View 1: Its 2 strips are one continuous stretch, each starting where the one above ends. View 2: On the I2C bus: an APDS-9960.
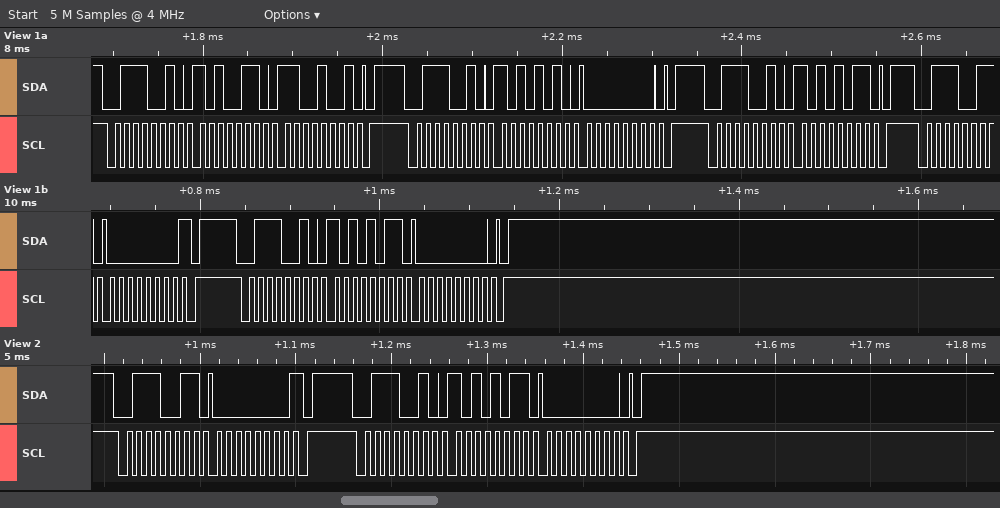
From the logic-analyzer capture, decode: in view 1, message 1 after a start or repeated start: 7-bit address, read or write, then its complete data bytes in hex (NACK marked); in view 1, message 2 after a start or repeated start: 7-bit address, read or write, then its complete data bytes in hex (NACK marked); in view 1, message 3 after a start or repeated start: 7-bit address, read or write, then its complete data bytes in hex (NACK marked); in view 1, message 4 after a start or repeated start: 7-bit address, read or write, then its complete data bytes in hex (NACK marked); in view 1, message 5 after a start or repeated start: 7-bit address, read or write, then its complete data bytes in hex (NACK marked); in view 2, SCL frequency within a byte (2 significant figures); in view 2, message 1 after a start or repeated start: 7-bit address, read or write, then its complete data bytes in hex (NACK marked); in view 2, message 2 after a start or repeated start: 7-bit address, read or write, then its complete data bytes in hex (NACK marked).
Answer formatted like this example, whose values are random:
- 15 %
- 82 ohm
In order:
- 0x39 write: A6 C9
- 0x39 write: AA 00
- 0x39 write: AB
- 0x39 read: 00 NACK
- 0x39 write: AB 00
- 100 kHz
- 0x39 read: 00 NACK
- 0x39 write: AB 00
